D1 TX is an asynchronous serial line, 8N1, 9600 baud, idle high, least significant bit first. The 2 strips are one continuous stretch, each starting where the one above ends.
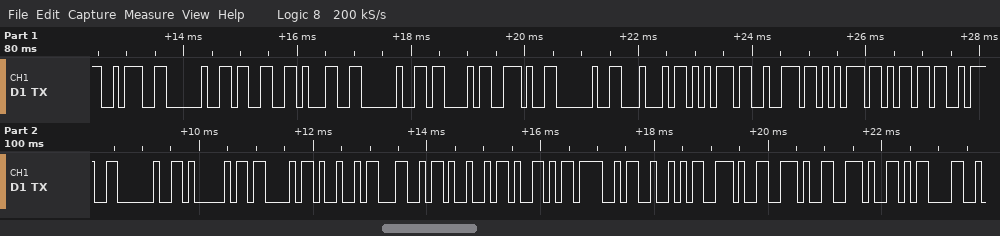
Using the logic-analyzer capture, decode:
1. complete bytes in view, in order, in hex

3A 20 33 31 20 43 2E 20 44 75 72 75 6D 3A 20 41 43 49 4C 49 59 4F 52 2E 2E 2E 0D
